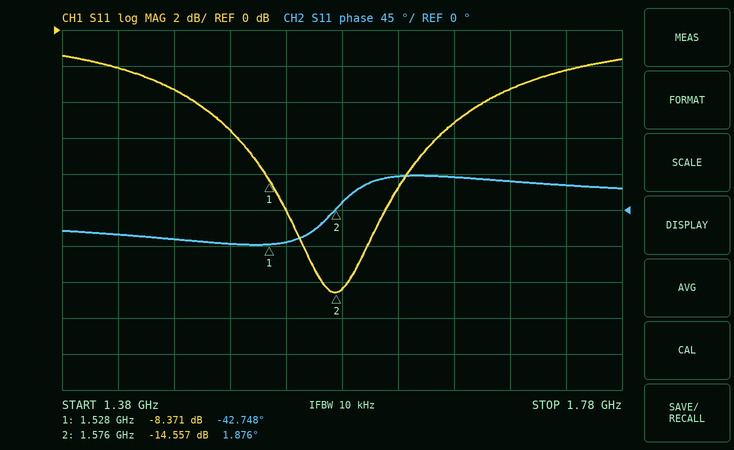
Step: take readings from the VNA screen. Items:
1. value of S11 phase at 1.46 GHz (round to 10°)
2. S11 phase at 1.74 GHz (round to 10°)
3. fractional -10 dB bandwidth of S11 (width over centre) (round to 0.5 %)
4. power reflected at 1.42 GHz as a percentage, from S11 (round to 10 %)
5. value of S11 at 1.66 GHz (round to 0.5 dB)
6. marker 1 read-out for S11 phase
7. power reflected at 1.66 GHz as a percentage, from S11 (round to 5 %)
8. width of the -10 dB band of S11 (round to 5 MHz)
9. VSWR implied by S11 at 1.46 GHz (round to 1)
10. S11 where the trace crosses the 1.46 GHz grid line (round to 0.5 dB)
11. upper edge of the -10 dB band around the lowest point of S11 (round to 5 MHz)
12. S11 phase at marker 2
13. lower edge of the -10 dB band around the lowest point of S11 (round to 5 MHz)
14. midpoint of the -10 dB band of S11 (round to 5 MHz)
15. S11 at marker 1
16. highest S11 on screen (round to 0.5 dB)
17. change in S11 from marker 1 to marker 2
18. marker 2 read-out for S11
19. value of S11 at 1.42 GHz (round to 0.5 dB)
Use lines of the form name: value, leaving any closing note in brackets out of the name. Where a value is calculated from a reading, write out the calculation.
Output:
value of S11 phase at 1.46 GHz: -40°
S11 phase at 1.74 GHz: 30°
fractional -10 dB bandwidth of S11 (width over centre): 70 MHz / 1.575 GHz ≈ 4.44 %, so 4.5 % to the nearest 0.5 %
power reflected at 1.42 GHz as a percentage, from S11: 10^(-2/10) ≈ 63.1 %, so 60 % to the nearest 10 %
value of S11 at 1.66 GHz: -5.0 dB
marker 1 read-out for S11 phase: -42.748°
power reflected at 1.66 GHz as a percentage, from S11: 10^(-5/10) ≈ 31.6 %, so 30 % to the nearest 5 %
width of the -10 dB band of S11: 1.610 GHz − 1.540 GHz = 70 MHz
VSWR implied by S11 at 1.46 GHz: |Γ| = 10^(-3.5/20) = 0.6683; VSWR = (1 + 0.6683)/(1 − 0.6683) ≈ 5
S11 where the trace crosses the 1.46 GHz grid line: -3.5 dB
upper edge of the -10 dB band around the lowest point of S11: 1.610 GHz
S11 phase at marker 2: 1.876°
lower edge of the -10 dB band around the lowest point of S11: 1.540 GHz
midpoint of the -10 dB band of S11: 1.575 GHz
S11 at marker 1: -8.371 dB
highest S11 on screen: -1.5 dB
change in S11 from marker 1 to marker 2: -14.557 − (-8.371) = -6.186 dB
marker 2 read-out for S11: -14.557 dB
value of S11 at 1.42 GHz: -2.0 dB
